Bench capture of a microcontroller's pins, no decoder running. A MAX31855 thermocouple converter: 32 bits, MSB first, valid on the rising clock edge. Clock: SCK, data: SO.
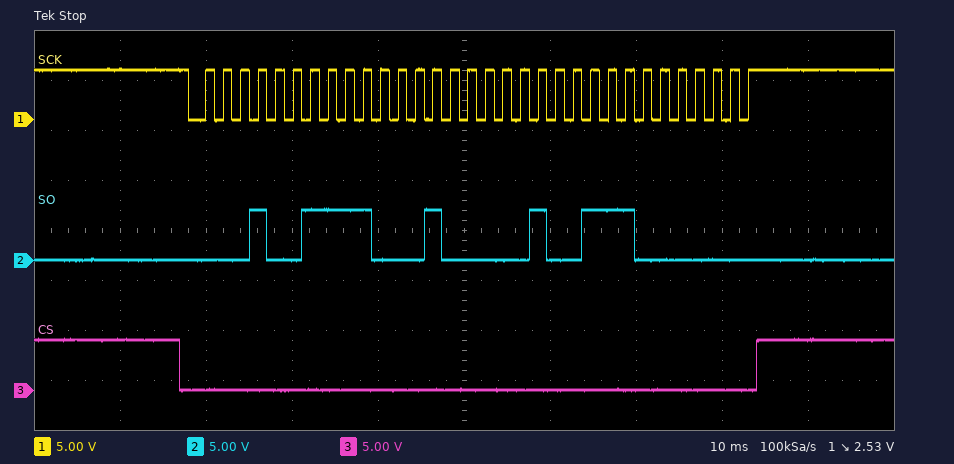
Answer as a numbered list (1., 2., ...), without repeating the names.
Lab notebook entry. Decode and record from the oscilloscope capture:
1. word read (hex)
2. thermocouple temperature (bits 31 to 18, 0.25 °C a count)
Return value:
1. 0x13C41380
2. 316.25 °C
